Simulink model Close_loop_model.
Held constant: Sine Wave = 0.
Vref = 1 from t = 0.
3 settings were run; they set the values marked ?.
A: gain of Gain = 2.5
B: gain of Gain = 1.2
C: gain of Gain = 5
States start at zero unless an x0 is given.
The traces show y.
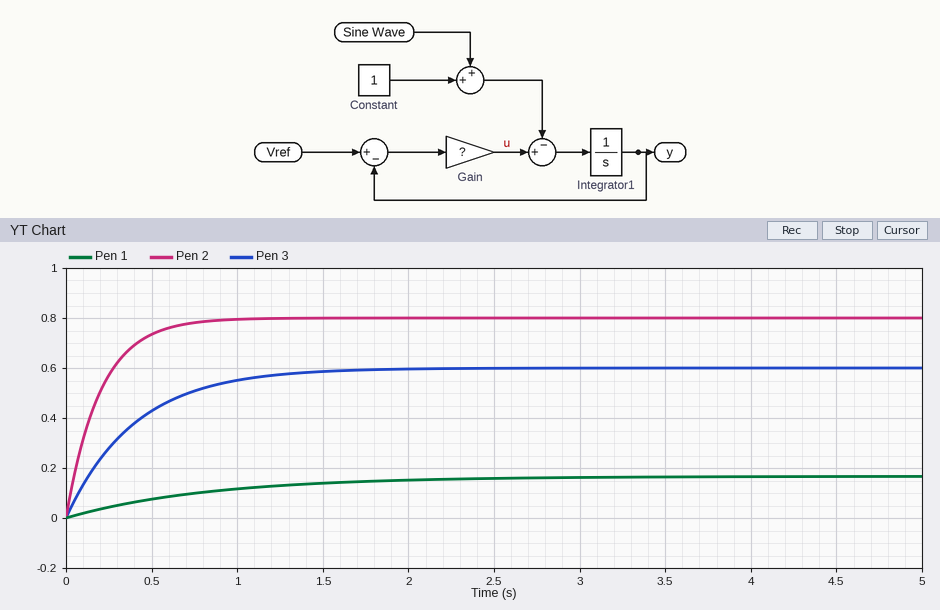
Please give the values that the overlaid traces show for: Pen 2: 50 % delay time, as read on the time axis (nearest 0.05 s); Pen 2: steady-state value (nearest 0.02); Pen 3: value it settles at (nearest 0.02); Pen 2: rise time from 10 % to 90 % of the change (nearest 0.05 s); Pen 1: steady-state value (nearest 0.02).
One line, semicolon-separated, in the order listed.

0.15 s; 0.80; 0.60; 0.45 s; 0.16
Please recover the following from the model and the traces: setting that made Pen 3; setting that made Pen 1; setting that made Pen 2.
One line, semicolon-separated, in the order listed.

A; B; C
